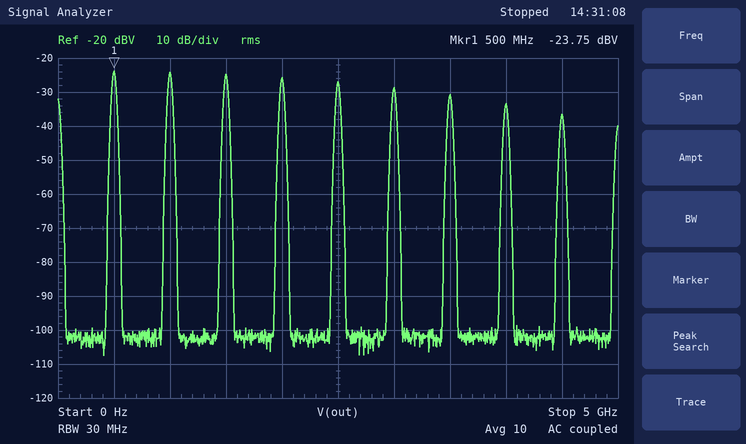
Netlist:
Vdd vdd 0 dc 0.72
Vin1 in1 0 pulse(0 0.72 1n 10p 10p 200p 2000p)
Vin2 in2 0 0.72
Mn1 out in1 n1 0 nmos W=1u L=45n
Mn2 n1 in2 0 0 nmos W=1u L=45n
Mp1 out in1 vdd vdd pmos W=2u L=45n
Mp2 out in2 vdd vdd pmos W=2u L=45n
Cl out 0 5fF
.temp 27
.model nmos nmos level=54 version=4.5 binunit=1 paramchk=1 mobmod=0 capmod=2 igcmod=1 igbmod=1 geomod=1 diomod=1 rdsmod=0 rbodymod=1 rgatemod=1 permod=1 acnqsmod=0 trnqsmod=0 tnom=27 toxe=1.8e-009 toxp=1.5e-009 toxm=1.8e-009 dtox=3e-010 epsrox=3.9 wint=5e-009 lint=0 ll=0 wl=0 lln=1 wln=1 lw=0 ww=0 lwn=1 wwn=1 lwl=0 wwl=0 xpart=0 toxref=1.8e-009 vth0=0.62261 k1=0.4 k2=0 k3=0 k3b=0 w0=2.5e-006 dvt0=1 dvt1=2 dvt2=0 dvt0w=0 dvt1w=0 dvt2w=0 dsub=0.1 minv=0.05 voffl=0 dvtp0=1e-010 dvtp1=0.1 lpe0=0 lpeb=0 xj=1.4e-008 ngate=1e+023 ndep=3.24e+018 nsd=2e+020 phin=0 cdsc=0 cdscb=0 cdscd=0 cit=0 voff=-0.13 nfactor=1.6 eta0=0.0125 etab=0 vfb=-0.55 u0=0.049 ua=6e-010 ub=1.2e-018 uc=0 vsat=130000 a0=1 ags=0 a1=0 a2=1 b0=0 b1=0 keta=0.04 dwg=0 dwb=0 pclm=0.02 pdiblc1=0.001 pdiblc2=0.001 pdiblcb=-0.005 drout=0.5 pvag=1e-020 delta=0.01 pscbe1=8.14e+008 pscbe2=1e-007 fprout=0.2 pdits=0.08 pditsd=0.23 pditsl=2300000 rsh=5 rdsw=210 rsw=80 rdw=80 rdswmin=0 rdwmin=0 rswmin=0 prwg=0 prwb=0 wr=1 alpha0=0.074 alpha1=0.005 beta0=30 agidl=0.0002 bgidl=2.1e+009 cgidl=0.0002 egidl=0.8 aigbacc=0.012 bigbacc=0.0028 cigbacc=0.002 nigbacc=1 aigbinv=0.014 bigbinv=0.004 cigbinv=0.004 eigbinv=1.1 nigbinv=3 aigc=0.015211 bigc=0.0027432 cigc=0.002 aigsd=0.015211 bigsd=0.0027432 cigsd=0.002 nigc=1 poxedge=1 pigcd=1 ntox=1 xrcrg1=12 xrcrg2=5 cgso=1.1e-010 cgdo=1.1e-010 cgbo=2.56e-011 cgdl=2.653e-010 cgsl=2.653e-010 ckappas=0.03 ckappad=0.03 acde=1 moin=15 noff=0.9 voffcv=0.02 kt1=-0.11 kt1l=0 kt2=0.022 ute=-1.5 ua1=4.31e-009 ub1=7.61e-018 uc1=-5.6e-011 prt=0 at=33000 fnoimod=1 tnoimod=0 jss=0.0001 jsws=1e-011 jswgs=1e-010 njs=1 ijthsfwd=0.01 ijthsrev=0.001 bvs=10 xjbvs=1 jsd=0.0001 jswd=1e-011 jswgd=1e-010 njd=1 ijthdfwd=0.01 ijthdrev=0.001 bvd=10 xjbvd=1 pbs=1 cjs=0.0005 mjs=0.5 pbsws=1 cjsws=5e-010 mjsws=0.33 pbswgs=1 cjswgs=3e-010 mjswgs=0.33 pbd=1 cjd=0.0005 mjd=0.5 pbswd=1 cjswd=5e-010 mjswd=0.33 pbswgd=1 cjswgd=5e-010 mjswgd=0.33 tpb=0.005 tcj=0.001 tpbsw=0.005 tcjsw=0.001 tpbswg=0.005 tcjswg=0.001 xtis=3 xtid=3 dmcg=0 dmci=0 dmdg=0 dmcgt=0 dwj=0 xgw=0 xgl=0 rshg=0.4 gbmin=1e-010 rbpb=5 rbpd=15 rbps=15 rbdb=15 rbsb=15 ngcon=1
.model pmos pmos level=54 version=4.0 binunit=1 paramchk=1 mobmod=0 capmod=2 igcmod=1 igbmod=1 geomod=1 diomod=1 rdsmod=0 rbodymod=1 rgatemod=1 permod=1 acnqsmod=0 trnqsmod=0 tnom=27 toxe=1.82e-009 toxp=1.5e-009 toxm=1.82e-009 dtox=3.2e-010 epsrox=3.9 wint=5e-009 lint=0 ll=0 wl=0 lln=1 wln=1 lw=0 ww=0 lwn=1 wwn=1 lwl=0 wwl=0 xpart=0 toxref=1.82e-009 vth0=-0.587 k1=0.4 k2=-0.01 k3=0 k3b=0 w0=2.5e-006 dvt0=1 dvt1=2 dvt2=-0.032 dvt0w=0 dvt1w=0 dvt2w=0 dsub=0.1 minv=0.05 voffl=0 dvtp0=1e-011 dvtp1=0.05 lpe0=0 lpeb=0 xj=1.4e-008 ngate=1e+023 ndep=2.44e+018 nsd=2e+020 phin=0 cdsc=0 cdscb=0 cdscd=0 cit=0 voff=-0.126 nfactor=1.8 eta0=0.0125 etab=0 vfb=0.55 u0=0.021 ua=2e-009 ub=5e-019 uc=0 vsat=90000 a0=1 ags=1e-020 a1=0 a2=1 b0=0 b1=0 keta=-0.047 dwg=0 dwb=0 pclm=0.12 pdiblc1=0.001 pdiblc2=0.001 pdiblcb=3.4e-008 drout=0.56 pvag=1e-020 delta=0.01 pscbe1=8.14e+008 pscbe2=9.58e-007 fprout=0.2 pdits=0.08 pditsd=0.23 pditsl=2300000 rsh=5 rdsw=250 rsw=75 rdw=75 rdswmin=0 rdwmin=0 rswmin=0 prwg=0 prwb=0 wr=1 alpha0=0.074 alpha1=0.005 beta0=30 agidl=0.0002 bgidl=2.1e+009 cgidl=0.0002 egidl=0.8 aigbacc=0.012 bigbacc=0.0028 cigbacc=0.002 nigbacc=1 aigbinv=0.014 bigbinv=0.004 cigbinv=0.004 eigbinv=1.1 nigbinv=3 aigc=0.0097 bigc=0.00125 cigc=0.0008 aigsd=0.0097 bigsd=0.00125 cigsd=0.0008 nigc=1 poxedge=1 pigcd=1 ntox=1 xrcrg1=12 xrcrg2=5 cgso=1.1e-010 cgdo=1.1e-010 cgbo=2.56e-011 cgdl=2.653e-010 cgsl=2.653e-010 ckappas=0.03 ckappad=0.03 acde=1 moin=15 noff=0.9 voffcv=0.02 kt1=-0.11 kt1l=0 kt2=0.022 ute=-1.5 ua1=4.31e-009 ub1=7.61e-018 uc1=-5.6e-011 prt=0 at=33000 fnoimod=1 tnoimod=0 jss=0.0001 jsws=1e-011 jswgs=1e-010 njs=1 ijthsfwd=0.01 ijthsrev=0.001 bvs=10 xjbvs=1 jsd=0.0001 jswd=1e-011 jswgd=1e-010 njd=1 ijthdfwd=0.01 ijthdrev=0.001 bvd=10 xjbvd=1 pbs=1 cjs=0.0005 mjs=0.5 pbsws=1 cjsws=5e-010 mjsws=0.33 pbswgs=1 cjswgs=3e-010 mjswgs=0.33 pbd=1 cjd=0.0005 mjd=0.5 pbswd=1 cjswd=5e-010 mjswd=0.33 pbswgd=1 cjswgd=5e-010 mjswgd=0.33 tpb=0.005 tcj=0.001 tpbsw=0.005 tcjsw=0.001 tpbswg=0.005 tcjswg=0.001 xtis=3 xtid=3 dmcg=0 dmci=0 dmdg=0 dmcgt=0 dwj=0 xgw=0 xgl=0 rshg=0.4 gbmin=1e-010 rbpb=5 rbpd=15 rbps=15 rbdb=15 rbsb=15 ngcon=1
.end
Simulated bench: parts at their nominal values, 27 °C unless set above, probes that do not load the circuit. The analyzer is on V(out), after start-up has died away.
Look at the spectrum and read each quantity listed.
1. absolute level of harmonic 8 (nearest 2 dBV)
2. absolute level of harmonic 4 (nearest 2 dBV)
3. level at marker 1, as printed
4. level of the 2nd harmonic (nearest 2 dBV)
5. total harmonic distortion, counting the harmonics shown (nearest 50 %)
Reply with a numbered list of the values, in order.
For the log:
1. -34 dBV
2. -26 dBV
3. -23.75 dBV
4. -24 dBV
5. 200 %
